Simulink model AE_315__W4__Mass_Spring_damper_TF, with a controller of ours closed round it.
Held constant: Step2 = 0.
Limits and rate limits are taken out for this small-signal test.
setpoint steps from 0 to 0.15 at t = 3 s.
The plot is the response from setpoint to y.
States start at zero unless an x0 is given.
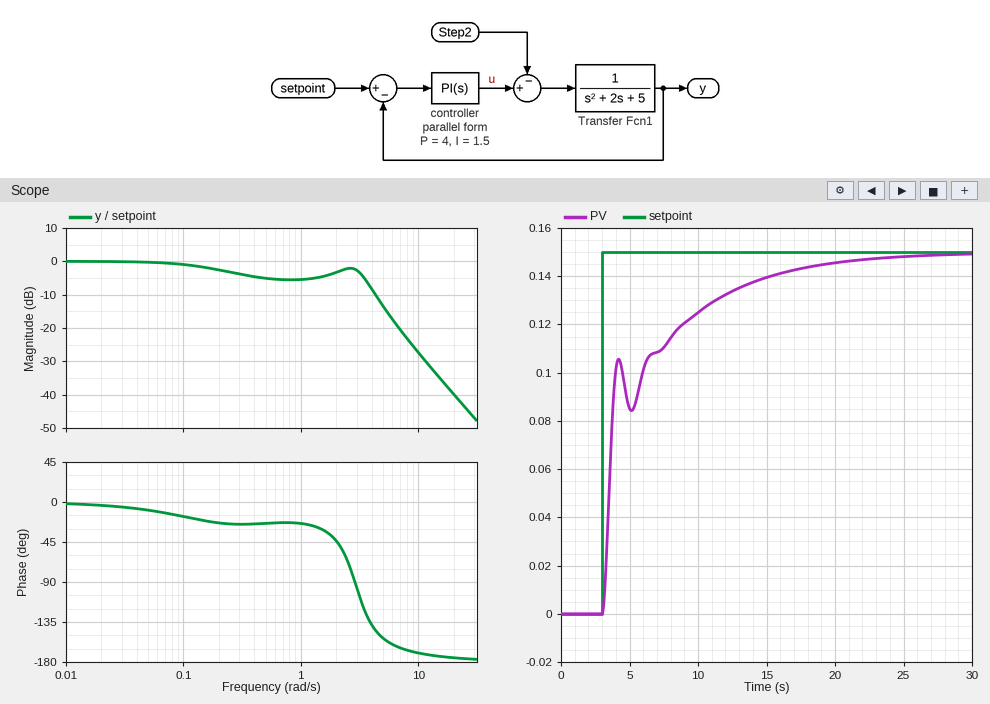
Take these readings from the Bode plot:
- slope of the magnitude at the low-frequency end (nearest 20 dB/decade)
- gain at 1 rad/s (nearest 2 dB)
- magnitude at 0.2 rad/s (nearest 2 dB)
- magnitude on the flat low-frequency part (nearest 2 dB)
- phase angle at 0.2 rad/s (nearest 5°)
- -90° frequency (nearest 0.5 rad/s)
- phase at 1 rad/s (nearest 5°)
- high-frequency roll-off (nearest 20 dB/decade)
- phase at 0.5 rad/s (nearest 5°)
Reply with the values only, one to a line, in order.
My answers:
0 dB/decade
-6 dB
-2 dB
0 dB
-25°
3.0 rad/s
-25°
-40 dB/decade
-25°
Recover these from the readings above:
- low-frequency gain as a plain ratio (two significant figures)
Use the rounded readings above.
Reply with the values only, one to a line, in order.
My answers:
1.0
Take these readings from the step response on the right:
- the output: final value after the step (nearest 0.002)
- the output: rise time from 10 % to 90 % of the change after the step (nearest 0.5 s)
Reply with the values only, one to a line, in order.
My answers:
0.150
9.5 s
